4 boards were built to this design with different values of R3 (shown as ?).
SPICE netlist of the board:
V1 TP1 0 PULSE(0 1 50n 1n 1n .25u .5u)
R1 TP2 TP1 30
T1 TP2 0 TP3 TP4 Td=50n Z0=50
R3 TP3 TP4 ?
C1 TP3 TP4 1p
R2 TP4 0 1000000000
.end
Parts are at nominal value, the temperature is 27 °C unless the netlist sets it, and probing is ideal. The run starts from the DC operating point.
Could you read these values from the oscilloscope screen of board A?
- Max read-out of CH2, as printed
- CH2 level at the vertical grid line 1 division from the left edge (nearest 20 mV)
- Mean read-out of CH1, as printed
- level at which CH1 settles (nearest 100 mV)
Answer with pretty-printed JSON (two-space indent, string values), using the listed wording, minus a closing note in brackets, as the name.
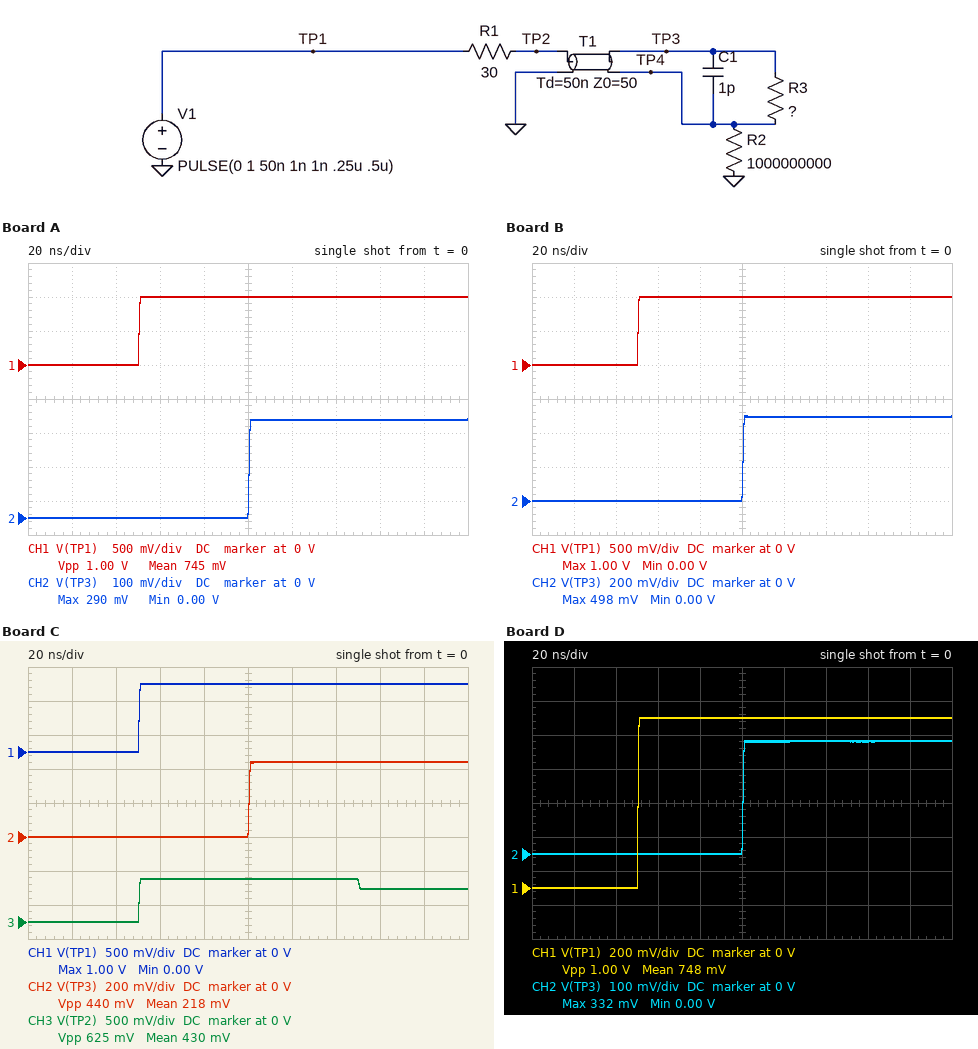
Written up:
{
  "Max read-out of CH2, as printed": "290 mV",
  "CH2 level at the vertical grid line 1 division from the left edge": "0 V",
  "Mean read-out of CH1, as printed": "745 mV",
  "level at which CH1 settles": "1.0 V"
}
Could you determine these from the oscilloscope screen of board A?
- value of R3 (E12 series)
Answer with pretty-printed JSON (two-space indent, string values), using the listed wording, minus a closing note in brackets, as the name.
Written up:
{
  "value of R3": "15 Ω"
}
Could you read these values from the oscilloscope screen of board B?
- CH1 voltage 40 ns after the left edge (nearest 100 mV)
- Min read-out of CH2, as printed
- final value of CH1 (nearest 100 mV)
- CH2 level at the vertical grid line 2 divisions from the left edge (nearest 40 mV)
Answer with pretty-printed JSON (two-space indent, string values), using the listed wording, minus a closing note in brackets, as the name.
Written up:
{
  "CH1 voltage 40 ns after the left edge": "0 V",
  "Min read-out of CH2, as printed": "0.00 V",
  "final value of CH1": "1.0 V",
  "CH2 level at the vertical grid line 2 divisions from the left edge": "0 V"
}
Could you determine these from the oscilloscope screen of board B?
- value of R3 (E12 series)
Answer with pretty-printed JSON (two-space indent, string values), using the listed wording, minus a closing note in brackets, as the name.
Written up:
{
  "value of R3": "33 Ω"
}
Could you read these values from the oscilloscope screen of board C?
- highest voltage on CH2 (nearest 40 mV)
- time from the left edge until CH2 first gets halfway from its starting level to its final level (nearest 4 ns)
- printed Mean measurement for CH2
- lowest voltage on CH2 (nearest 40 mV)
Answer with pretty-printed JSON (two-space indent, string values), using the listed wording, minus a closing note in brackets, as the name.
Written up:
{
  "highest voltage on CH2": "440 mV",
  "time from the left edge until CH2 first gets halfway from its starting level to its final level": "100 ns",
  "printed Mean measurement for CH2": "218 mV",
  "lowest voltage on CH2": "0 V"
}
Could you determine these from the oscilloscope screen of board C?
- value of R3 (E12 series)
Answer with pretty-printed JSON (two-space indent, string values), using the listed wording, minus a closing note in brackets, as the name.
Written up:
{
  "value of R3": "27 Ω"
}
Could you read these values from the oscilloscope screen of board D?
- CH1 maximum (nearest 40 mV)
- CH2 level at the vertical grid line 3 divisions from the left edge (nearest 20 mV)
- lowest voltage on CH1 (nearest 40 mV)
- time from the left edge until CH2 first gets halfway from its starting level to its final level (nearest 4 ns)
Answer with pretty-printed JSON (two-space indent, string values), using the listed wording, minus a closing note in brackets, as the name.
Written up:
{
  "CH1 maximum": "1.00 V",
  "CH2 level at the vertical grid line 3 divisions from the left edge": "0 V",
  "lowest voltage on CH1": "0 V",
  "time from the left edge until CH2 first gets halfway from its starting level to its final level": "100 ns"
}
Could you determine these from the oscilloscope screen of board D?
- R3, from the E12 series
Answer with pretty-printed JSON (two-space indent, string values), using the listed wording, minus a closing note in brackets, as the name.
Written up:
{
  "R3, from the E12 series": "18 Ω"
}
